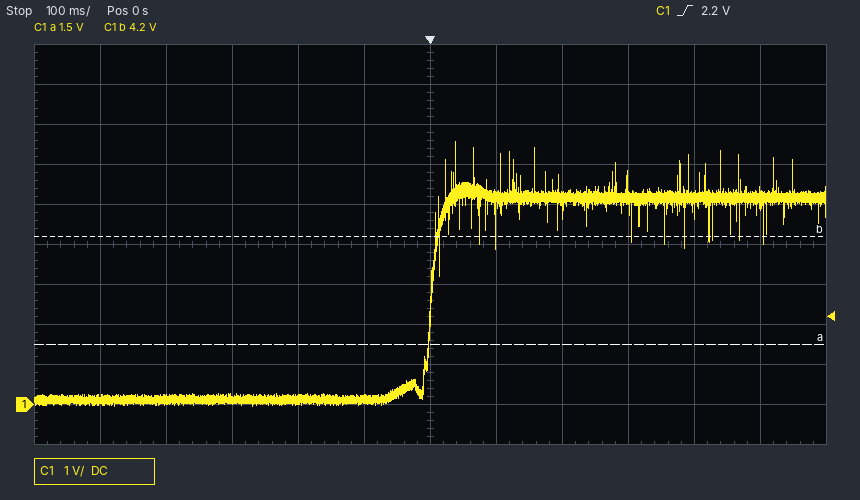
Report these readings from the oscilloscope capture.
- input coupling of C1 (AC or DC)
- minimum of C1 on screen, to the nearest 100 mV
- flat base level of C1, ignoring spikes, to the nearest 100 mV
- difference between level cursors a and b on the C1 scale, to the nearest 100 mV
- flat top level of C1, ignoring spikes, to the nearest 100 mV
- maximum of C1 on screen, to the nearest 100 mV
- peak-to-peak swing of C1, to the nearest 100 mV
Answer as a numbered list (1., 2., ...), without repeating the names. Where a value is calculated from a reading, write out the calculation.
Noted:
1. DC
2. 0.0 V
3. 100 mV
4. 2.7 V
5. 5.2 V
6. 6.6 V
7. 6.6 V − (0.0 V) = 6.6 V
